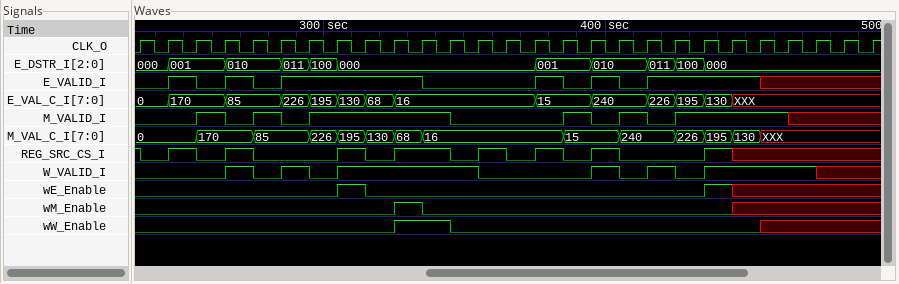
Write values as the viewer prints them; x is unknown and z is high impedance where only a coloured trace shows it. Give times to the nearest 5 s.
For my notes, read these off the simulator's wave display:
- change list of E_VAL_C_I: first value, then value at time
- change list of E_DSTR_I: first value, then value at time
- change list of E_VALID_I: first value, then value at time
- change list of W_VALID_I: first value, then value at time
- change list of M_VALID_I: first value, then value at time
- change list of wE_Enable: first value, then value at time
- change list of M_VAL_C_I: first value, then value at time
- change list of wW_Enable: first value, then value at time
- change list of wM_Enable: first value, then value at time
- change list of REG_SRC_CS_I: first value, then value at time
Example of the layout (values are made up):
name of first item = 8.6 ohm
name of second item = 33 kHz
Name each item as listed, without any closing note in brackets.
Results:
change list of E_VAL_C_I: first value, then value at time = 0, 170 at 245 s, 85 at 265 s, 226 at 285 s, 195 at 295 s, 130 at 305 s, 68 at 315 s, 16 at 325 s, 15 at 375 s, 240 at 395 s, 226 at 415 s, 195 at 425 s, 130 at 435 s, XXX at 445 s
change list of E_DSTR_I: first value, then value at time = 000, 001 at 245 s, 010 at 265 s, 011 at 285 s, 100 at 295 s, 000 at 305 s, 001 at 375 s, 010 at 395 s, 011 at 415 s, 100 at 425 s, 000 at 435 s
change list of E_VALID_I: first value, then value at time = 0, 1 at 245 s, 0 at 255 s, 1 at 265 s, 0 at 275 s, 1 at 285 s, 0 at 335 s, 1 at 375 s, 0 at 385 s, 1 at 395 s, 0 at 405 s, 1 at 415 s, x at 455 s
change list of W_VALID_I: first value, then value at time = 0, 1 at 265 s, 0 at 275 s, 1 at 285 s, 0 at 295 s, 1 at 305 s, 0 at 355 s, 1 at 395 s, 0 at 405 s, 1 at 415 s, 0 at 425 s, 1 at 435 s, x at 475 s
change list of M_VALID_I: first value, then value at time = 0, 1 at 255 s, 0 at 265 s, 1 at 275 s, 0 at 285 s, 1 at 295 s, 0 at 345 s, 1 at 385 s, 0 at 395 s, 1 at 405 s, 0 at 415 s, 1 at 425 s, x at 465 s
change list of wE_Enable: first value, then value at time = 0, 1 at 305 s, 0 at 315 s, 1 at 435 s, x at 445 s
change list of M_VAL_C_I: first value, then value at time = 0, 170 at 255 s, 85 at 275 s, 226 at 295 s, 195 at 305 s, 130 at 315 s, 68 at 325 s, 16 at 335 s, 15 at 385 s, 240 at 405 s, 226 at 425 s, 195 at 435 s, 130 at 445 s, XXX at 455 s
change list of wW_Enable: first value, then value at time = 0, 1 at 325 s, 0 at 345 s, x at 455 s
change list of wM_Enable: first value, then value at time = 0, 1 at 325 s, 0 at 335 s, x at 445 s
change list of REG_SRC_CS_I: first value, then value at time = 1, 0 at 235 s, 1 at 245 s, 0 at 255 s, 1 at 265 s, 0 at 275 s, 1 at 305 s, 0 at 315 s, 1 at 325 s, 0 at 345 s, 1 at 355 s, 0 at 365 s, 1 at 375 s, 0 at 385 s, 1 at 395 s, 0 at 405 s, 1 at 435 s, x at 445 s
